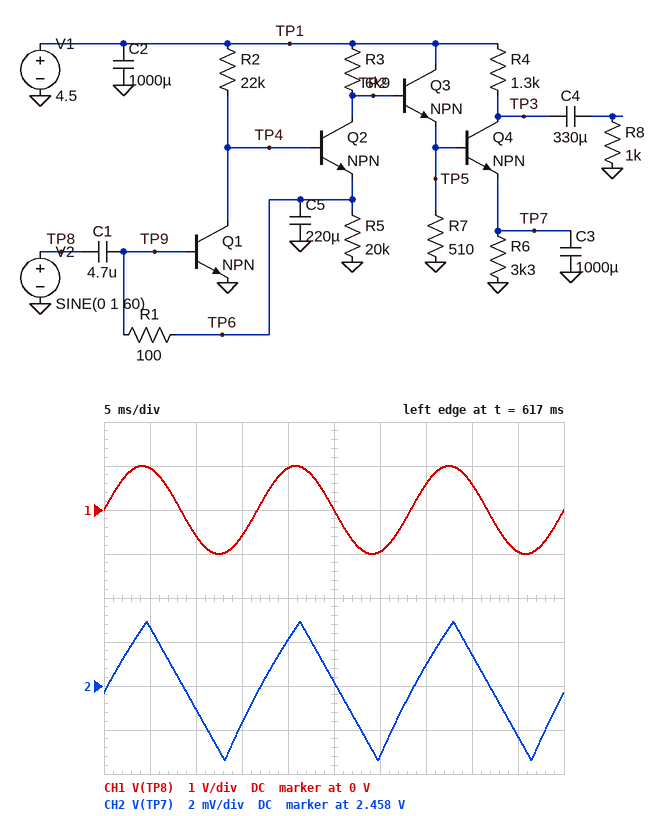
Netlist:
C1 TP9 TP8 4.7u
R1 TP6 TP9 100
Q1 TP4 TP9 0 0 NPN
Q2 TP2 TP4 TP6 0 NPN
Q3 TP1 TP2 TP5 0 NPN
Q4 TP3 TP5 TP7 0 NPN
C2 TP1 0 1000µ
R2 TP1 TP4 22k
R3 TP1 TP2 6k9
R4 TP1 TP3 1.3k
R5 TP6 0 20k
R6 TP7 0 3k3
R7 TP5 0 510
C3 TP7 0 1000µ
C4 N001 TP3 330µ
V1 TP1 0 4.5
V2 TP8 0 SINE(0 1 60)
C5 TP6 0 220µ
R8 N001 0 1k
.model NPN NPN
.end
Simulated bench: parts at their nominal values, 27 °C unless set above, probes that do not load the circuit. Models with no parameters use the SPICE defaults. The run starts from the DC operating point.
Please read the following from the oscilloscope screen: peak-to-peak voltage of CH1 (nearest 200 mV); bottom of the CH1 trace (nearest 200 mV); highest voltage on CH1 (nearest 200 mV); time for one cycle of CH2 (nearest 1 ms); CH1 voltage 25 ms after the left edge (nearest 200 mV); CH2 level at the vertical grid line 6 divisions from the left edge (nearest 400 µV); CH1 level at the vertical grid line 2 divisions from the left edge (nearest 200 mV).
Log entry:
2.0 V
-1.0 V
1.0 V
17 ms
0 V
2.4548 V
-600 mV
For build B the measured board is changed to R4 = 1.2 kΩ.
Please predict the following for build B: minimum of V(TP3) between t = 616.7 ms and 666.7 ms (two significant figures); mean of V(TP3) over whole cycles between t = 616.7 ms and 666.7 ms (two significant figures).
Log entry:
3.1 V
3.6 V
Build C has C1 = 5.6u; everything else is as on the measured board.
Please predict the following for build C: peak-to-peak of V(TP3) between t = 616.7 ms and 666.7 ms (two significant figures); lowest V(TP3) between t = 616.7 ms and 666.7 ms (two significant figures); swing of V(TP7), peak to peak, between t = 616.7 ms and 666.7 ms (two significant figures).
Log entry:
1.0 V
2.9 V
6.6 mV
